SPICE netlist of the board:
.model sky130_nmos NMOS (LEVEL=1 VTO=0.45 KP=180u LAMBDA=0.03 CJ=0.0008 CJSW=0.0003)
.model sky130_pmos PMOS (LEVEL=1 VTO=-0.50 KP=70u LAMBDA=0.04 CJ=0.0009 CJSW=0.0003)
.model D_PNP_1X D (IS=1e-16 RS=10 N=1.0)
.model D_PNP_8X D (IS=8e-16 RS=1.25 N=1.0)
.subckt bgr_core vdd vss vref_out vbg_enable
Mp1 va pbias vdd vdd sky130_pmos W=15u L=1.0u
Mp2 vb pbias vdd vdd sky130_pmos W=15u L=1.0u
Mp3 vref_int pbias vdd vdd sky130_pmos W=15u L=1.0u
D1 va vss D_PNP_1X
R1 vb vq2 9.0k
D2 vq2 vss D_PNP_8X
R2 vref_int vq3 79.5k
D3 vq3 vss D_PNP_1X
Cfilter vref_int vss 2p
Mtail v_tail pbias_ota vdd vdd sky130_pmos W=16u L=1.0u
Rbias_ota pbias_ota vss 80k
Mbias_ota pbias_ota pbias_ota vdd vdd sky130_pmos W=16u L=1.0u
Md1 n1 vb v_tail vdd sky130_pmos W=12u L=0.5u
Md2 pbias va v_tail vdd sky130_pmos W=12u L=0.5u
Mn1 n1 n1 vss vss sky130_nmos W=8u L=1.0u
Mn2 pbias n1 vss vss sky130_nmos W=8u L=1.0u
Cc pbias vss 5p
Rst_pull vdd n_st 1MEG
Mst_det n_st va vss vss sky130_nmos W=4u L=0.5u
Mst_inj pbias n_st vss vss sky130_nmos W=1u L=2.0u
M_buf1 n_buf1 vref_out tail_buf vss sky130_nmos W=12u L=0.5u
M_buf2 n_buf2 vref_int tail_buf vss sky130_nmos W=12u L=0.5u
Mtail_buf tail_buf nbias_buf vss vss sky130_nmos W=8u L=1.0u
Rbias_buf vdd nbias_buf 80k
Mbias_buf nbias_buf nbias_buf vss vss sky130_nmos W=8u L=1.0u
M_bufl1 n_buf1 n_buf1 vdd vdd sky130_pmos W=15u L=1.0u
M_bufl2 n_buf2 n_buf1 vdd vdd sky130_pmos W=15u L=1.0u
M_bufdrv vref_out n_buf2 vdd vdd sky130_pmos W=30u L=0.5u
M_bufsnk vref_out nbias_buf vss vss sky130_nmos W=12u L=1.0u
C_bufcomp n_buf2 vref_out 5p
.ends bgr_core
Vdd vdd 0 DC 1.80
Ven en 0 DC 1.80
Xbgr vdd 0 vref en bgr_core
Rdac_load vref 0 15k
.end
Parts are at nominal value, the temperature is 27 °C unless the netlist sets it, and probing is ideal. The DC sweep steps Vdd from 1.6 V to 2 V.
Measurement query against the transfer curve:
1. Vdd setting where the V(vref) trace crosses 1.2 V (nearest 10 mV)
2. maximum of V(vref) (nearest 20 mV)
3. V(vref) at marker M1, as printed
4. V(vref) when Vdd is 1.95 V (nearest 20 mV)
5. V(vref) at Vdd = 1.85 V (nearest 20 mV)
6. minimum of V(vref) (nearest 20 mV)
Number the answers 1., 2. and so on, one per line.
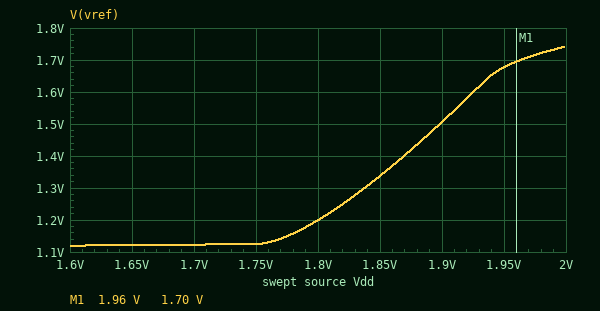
1. 1.80 V
2. 1.74 V
3. 1.70 V
4. 1.68 V
5. 1.34 V
6. 1.12 V
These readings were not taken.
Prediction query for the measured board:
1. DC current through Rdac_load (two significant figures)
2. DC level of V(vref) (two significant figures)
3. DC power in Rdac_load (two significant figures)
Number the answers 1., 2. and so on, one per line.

1. 80 µA
2. 1.2 V
3. 96 µW
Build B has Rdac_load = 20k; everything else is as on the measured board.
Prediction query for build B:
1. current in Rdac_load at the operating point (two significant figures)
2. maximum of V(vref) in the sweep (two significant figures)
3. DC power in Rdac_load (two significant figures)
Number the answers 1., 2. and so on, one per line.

1. 60 µA
2. 1.8 V
3. 72 µW
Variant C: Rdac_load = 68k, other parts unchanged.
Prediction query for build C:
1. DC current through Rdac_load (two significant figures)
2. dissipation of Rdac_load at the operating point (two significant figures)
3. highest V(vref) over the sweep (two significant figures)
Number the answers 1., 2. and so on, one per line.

1. 18 µA
2. 21 µW
3. 1.8 V
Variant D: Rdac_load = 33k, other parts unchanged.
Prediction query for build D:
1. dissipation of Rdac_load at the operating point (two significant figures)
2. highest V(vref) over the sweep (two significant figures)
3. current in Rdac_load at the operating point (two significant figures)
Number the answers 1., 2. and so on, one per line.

1. 44 µW
2. 1.8 V
3. 36 µA
